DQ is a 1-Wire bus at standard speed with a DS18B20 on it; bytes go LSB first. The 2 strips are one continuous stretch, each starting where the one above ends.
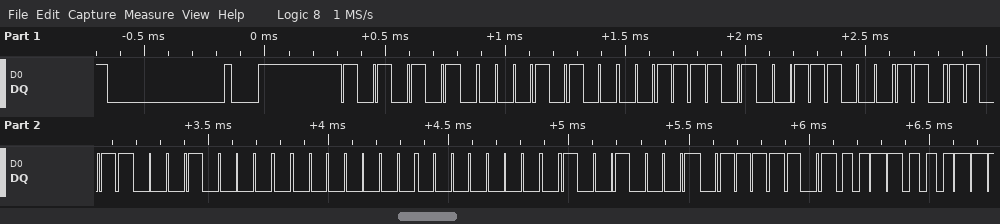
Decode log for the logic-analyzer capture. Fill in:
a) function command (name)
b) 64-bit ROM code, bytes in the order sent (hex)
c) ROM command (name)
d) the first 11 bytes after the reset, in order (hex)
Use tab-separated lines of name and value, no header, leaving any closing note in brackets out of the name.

function command	Read Scratchpad
64-bit ROM code, bytes in the order sent	28 BC 1C DB 08 00 00 89
ROM command	Match ROM
the first 11 bytes after the reset, in order	55 28 BC 1C DB 08 00 00 89 BE 8C
